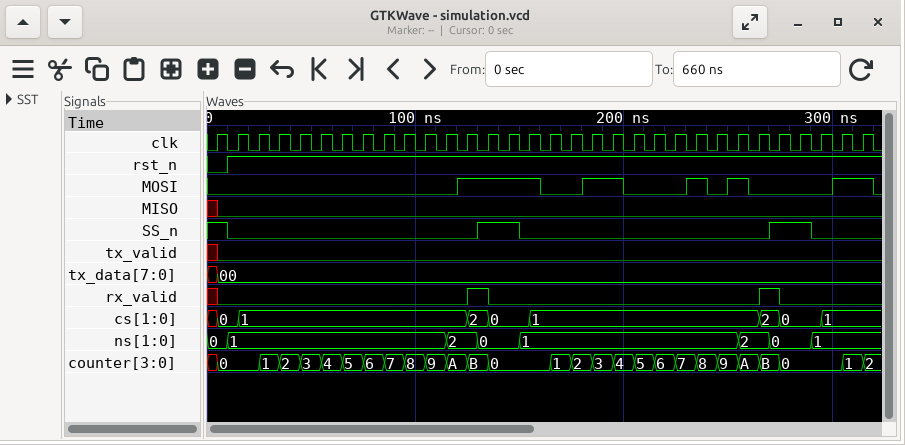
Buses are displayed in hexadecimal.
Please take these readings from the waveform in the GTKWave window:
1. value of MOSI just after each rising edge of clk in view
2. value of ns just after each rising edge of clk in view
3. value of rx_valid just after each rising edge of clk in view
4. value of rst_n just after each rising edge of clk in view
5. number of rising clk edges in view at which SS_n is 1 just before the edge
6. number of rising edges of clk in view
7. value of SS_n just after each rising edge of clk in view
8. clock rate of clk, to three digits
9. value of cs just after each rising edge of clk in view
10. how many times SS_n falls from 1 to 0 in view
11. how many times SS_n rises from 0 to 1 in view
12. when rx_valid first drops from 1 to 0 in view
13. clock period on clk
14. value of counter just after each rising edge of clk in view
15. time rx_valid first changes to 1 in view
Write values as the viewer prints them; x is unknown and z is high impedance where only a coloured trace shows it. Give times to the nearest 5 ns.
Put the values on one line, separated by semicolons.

0 0 0 0 0 0 0 0 0 0 0 0 1 1 1 1 0 0 1 1 0 0 0 1 0 1 0 0 0 0 1 1; 0, 1, 1, 1, 1, 1, 1, 1, 1, 1, 1, 2, 2, 0, 0, 1, 1, 1, 1, 1, 1, 1, 1, 1, 1, 2, 2, 0, 0, 1, 1, 1; 0 0 0 0 0 0 0 0 0 0 0 0 1 0 0 0 0 0 0 0 0 0 0 0 0 0 1 0 0 0 0 0; 0 1 1 1 1 1 1 1 1 1 1 1 1 1 1 1 1 1 1 1 1 1 1 1 1 1 1 1 1 1 1 1; 5; 32; 1 0 0 0 0 0 0 0 0 0 0 0 0 1 1 0 0 0 0 0 0 0 0 0 0 0 0 1 1 0 0 0; 100 MHz; 0, 1, 1, 1, 1, 1, 1, 1, 1, 1, 1, 1, 2, 0, 0, 1, 1, 1, 1, 1, 1, 1, 1, 1, 1, 1, 2, 0, 0, 1, 1, 1; 3; 2; 135 ns; 10 ns; 0, 0, 1, 2, 3, 4, 5, 6, 7, 8, 9, A, B, 0, 0, 0, 1, 2, 3, 4, 5, 6, 7, 8, 9, A, B, 0, 0, 0, 1, 2; 125 ns
